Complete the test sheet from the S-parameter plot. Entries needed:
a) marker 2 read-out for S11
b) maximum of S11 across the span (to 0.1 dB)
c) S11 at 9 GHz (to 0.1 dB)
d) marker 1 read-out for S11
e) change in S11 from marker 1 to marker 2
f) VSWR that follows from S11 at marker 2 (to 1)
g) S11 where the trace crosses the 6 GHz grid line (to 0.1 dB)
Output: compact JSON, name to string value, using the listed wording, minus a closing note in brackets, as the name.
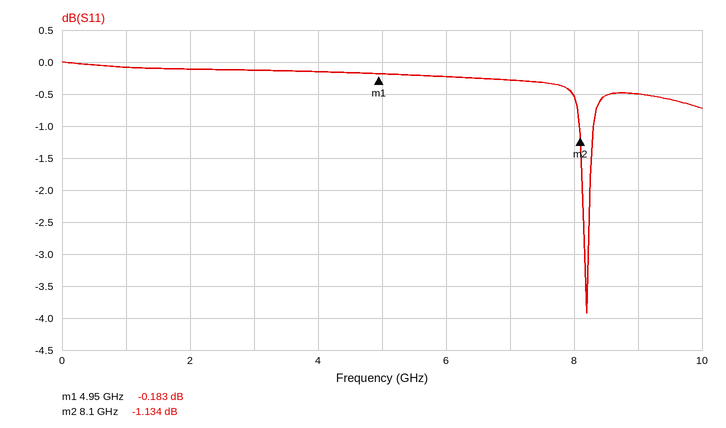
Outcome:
{"marker 2 read-out for S11": "-1.134 dB", "maximum of S11 across the span": "0.0 dB", "S11 at 9 GHz": "-0.5 dB", "marker 1 read-out for S11": "-0.183 dB", "change in S11 from marker 1 to marker 2": "-0.951 dB", "VSWR that follows from S11 at marker 2": "15", "S11 where the trace crosses the 6 GHz grid line": "-0.2 dB"}
